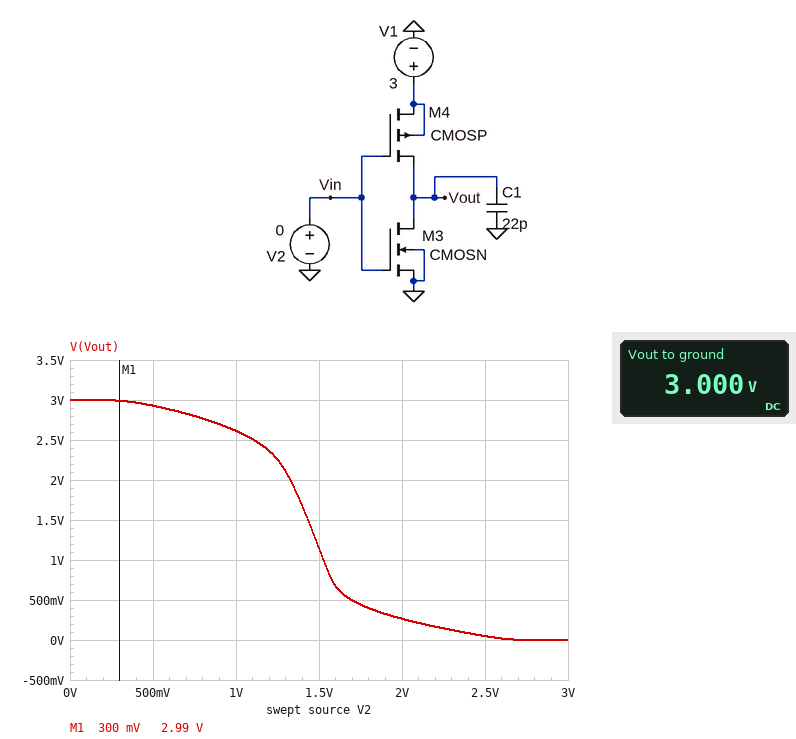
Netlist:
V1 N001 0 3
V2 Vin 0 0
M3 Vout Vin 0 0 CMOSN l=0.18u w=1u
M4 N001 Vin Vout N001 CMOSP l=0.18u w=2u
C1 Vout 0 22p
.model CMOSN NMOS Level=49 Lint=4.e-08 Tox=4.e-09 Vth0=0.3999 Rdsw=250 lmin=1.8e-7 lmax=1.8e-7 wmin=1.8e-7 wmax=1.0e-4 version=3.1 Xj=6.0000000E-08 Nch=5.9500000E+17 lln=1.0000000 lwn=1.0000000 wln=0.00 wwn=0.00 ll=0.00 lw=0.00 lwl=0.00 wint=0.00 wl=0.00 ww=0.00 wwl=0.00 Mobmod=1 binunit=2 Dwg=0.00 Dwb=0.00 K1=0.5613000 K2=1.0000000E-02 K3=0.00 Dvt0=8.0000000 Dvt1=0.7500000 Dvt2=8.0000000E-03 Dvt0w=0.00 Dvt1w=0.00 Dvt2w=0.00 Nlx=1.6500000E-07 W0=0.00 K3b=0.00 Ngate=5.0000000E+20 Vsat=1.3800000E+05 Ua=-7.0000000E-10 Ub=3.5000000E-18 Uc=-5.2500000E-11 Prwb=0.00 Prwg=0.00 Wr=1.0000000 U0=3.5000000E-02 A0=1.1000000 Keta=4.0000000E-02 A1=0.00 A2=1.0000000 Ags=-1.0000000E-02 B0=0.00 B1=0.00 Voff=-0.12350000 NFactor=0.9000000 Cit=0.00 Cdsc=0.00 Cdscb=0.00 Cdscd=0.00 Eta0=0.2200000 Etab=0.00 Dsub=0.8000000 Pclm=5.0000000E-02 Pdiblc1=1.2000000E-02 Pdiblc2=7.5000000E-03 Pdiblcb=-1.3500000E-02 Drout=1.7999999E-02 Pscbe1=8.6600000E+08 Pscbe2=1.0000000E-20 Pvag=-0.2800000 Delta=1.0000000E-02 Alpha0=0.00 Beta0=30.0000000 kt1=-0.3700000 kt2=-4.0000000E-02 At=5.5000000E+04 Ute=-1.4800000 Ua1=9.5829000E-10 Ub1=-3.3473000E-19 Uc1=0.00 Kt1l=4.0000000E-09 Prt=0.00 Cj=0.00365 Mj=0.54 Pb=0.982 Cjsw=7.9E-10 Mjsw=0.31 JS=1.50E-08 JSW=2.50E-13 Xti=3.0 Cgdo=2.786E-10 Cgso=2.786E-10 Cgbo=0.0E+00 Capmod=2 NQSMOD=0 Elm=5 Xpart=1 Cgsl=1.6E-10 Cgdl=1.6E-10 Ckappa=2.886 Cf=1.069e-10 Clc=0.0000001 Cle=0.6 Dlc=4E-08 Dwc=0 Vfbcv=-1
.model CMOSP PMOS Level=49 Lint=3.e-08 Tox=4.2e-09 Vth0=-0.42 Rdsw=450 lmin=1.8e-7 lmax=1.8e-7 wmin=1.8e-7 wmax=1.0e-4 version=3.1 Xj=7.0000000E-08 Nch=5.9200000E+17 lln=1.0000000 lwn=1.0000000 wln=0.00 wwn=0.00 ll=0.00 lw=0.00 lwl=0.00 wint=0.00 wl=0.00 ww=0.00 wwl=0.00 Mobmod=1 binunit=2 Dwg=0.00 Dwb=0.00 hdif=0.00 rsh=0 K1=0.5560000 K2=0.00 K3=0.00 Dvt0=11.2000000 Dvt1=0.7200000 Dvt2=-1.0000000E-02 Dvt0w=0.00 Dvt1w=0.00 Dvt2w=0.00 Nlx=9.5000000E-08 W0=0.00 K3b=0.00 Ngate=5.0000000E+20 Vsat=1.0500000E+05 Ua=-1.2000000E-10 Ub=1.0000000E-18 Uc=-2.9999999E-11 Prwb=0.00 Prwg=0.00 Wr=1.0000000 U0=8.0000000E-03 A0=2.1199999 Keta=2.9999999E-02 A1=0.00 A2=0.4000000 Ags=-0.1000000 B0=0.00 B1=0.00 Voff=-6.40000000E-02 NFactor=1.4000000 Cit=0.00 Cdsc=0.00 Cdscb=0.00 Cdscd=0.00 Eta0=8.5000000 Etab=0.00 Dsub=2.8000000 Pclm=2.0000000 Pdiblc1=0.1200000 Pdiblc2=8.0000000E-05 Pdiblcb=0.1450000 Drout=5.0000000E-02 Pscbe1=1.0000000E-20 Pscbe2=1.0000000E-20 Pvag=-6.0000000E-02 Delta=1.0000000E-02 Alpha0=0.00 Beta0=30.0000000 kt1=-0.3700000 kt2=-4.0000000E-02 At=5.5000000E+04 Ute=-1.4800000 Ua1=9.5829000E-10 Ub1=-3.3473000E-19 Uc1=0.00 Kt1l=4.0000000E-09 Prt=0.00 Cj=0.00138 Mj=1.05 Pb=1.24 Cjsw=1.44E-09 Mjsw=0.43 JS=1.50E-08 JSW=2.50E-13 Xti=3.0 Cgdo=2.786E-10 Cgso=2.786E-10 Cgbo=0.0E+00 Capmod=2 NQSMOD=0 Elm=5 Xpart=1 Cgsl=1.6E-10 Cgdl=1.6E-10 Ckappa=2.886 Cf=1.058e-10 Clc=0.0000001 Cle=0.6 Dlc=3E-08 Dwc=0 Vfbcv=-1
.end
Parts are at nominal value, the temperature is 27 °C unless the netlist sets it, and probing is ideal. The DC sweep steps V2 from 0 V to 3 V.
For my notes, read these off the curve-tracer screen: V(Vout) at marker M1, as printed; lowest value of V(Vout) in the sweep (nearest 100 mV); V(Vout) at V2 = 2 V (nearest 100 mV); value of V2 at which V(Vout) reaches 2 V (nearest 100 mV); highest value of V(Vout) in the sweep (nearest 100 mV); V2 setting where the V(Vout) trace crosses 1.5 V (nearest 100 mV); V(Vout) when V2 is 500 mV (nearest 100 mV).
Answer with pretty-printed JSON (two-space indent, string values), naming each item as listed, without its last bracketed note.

{
  "V(Vout) at marker M1, as printed": "2.99 V",
  "lowest value of V(Vout) in the sweep": "0 V",
  "V(Vout) at V2 = 2 V": "300 mV",
  "value of V2 at which V(Vout) reaches 2 V": "1.3 V",
  "highest value of V(Vout) in the sweep": "3.0 V",
  "V2 setting where the V(Vout) trace crosses 1.5 V": "1.4 V",
  "V(Vout) when V2 is 500 mV": "2.9 V"
}
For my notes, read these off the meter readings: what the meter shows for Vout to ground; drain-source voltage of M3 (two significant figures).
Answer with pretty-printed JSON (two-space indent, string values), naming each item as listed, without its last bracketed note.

{
  "what the meter shows for Vout to ground": "3.000 V",
  "drain-source voltage of M3": "3.0 V"
}
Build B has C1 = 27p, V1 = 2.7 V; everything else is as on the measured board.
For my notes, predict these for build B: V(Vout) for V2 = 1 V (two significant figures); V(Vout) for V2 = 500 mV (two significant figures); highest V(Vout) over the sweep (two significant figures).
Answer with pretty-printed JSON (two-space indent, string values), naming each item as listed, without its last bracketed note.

{
  "V(Vout) for V2 = 1 V": "2.3 V",
  "V(Vout) for V2 = 500 mV": "2.6 V",
  "highest V(Vout) over the sweep": "2.7 V"
}
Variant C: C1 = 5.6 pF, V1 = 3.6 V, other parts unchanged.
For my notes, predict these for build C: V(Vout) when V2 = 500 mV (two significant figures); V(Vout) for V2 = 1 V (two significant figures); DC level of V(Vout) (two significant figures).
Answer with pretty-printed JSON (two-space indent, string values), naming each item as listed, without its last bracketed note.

{
  "V(Vout) when V2 = 500 mV": "3.5 V",
  "V(Vout) for V2 = 1 V": "3.2 V",
  "DC level of V(Vout)": "3.6 V"
}
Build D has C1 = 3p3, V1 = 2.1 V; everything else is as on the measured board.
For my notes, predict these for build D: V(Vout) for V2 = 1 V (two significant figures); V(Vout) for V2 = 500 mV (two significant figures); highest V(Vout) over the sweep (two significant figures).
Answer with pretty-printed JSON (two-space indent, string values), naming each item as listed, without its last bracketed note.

{
  "V(Vout) for V2 = 1 V": "1.1 V",
  "V(Vout) for V2 = 500 mV": "2.0 V",
  "highest V(Vout) over the sweep": "2.1 V"
}
